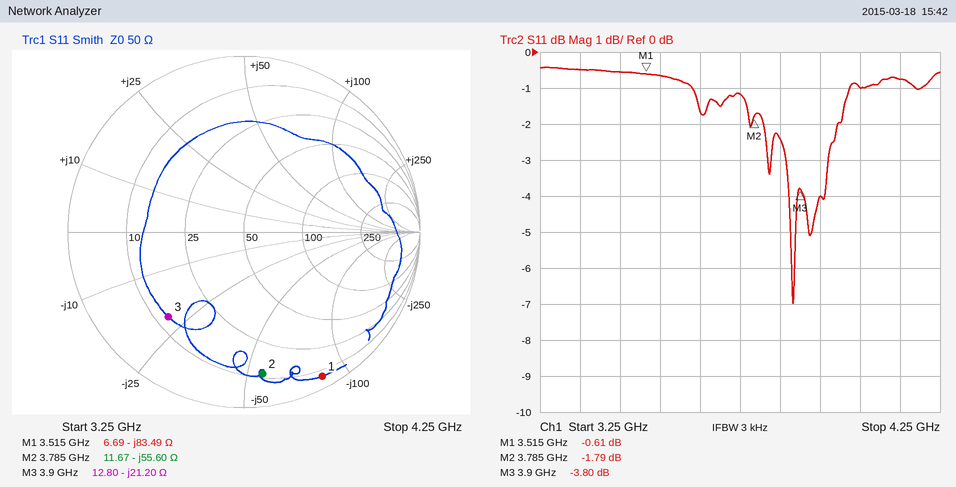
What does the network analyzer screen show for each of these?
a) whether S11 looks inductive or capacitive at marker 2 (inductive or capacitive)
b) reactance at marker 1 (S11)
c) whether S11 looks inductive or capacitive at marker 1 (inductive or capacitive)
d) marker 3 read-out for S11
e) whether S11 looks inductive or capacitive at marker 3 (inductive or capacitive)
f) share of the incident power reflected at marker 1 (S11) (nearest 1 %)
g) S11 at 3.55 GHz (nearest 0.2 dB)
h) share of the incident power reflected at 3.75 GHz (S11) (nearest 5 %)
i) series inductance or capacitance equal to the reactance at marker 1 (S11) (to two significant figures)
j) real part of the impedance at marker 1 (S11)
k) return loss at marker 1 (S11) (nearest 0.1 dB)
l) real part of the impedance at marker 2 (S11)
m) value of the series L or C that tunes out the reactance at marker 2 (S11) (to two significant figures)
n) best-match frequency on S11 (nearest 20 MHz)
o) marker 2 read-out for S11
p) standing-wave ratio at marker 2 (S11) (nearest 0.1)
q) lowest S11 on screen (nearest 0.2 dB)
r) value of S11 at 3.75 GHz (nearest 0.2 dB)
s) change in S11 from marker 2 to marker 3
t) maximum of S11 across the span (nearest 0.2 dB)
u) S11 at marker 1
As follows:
capacitive
-83.49 Ω
capacitive
-3.80 dB
capacitive
87 %
-0.6 dB
75 %
540 fF
6.69 Ω
0.6 dB
11.67 Ω
2.3 nH
3.88 GHz
-1.79 dB
9.7
-7.0 dB
-1.2 dB
-2.01 dB
-0.4 dB
-0.61 dB
